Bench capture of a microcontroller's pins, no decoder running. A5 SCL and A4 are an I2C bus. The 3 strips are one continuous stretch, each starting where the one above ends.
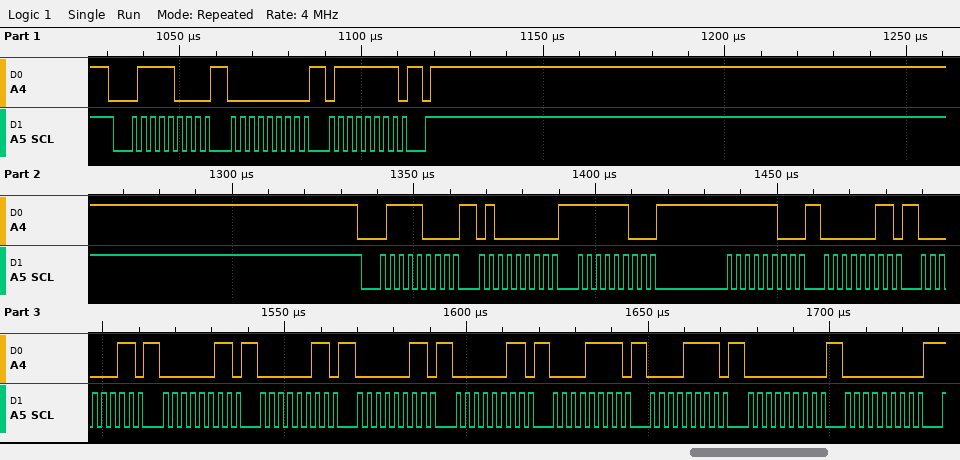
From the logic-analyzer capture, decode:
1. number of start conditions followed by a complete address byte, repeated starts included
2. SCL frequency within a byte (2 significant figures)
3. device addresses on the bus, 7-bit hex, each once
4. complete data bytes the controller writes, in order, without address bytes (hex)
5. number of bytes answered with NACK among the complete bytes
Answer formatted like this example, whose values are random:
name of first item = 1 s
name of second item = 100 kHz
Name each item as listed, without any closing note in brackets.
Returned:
number of start conditions followed by a complete address byte, repeated starts included = 2
SCL frequency within a byte = 400 kHz
device addresses on the bus, 7-bit hex, each once = 0x3C
complete data bytes the controller writes, in order, without address bytes = 00 7F 40 FC FC 03 03 03 03 03 03 0F 0F 00 00
number of bytes answered with NACK among the complete bytes = 0
